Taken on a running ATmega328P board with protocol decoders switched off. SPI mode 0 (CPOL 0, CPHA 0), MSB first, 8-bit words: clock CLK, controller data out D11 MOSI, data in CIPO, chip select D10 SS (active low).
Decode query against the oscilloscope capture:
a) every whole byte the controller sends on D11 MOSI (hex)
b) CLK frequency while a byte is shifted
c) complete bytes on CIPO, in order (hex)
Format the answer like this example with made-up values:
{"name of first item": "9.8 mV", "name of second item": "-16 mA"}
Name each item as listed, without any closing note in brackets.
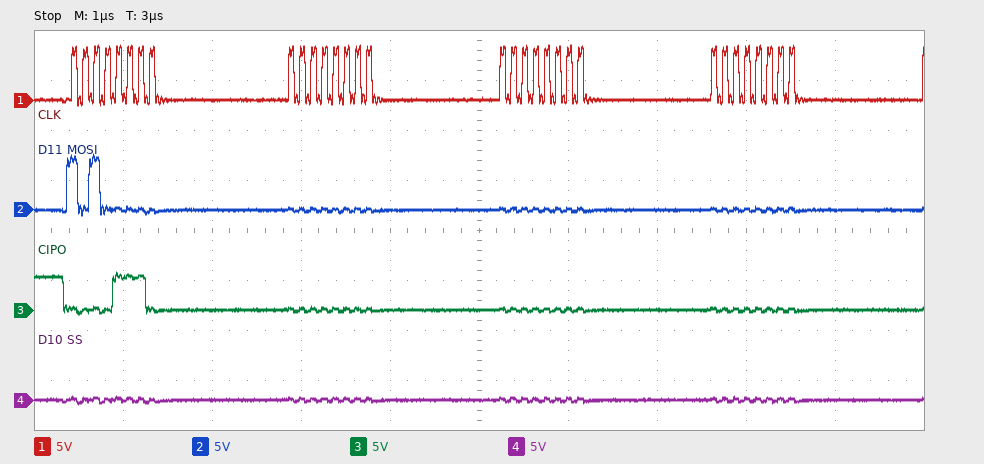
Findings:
{"every whole byte the controller sends on D11 MOSI": "A0 00 00 00", "CLK frequency while a byte is shifted": "8 MHz", "complete bytes on CIPO, in order": "0E 00 00 00"}
